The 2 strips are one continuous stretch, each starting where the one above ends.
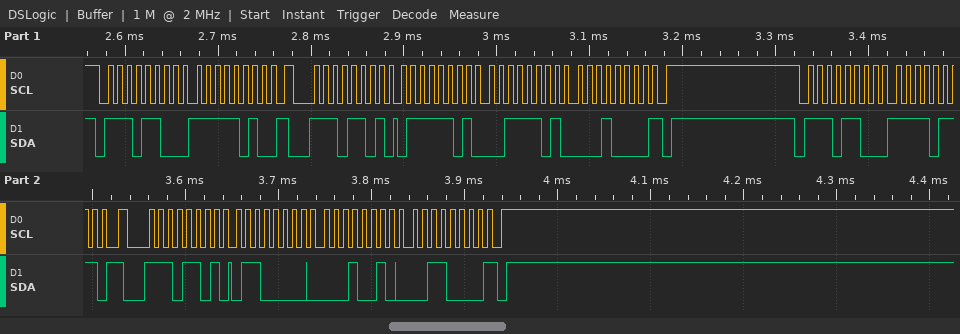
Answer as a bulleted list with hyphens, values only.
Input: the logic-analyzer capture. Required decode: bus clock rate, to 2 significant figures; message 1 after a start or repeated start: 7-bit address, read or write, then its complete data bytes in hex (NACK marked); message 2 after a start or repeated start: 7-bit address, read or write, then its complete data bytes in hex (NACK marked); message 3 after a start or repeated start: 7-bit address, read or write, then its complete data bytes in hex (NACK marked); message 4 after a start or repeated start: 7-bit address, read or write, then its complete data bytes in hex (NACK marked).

- 100 kHz
- 0x76 write: FA
- 0x76 read: 7D 3D 10 NACK
- 0x76 write: F7
- 0x76 read: 60 12 30 NACK
